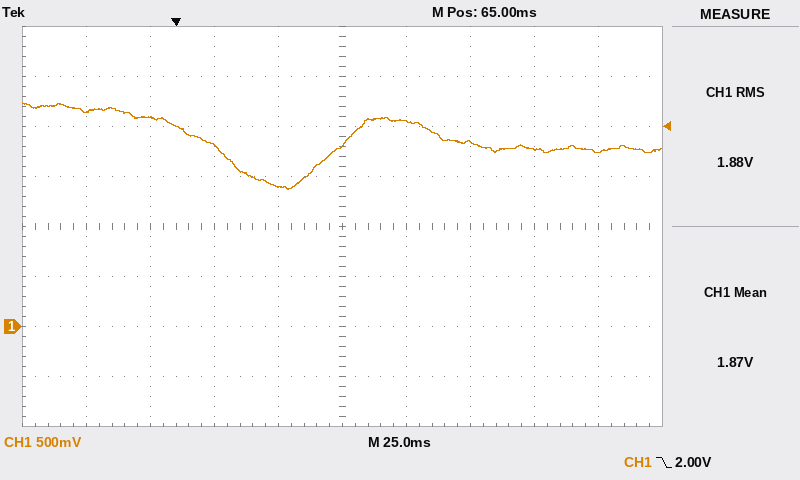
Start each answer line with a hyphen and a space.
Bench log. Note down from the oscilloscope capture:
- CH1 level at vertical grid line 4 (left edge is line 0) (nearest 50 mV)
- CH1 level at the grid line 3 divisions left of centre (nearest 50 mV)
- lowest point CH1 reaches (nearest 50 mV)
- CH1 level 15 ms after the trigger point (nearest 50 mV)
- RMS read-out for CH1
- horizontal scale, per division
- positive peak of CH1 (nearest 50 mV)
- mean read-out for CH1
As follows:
- 1.40 V
- 2.10 V
- 1.35 V
- 1.80 V
- 1.88 V
- 25 ms
- 2.25 V
- 1.87 V
